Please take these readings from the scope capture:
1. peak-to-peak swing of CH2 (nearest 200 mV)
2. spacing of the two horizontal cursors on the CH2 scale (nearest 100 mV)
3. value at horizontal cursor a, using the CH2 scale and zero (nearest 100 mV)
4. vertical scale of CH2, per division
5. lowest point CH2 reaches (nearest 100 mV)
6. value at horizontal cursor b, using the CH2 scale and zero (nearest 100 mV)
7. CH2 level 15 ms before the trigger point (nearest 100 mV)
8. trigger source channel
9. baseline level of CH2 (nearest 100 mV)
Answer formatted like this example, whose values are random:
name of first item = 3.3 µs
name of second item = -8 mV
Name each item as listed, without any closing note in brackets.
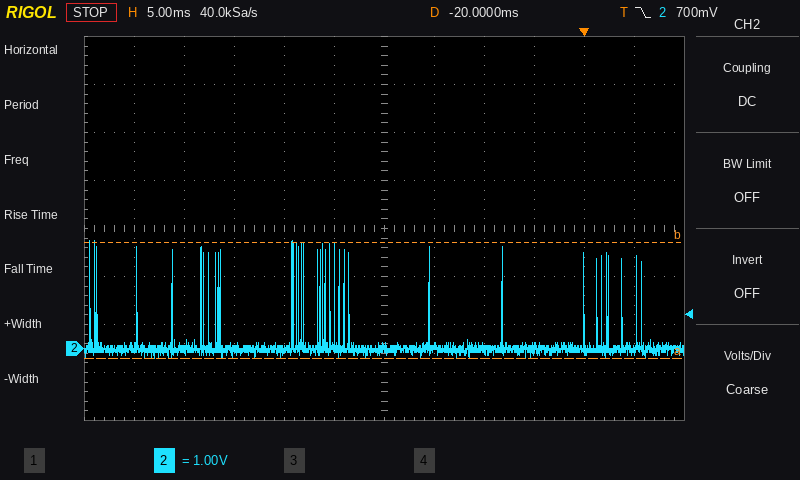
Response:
peak-to-peak swing of CH2 = 2.4 V
spacing of the two horizontal cursors on the CH2 scale = 2.4 V
value at horizontal cursor a, using the CH2 scale and zero = -200 mV
vertical scale of CH2, per division = 1 V
lowest point CH2 reaches = -200 mV
value at horizontal cursor b, using the CH2 scale and zero = 2.2 V
CH2 level 15 ms before the trigger point = 0.0 V
trigger source channel = CH2
baseline level of CH2 = 0.0 V
